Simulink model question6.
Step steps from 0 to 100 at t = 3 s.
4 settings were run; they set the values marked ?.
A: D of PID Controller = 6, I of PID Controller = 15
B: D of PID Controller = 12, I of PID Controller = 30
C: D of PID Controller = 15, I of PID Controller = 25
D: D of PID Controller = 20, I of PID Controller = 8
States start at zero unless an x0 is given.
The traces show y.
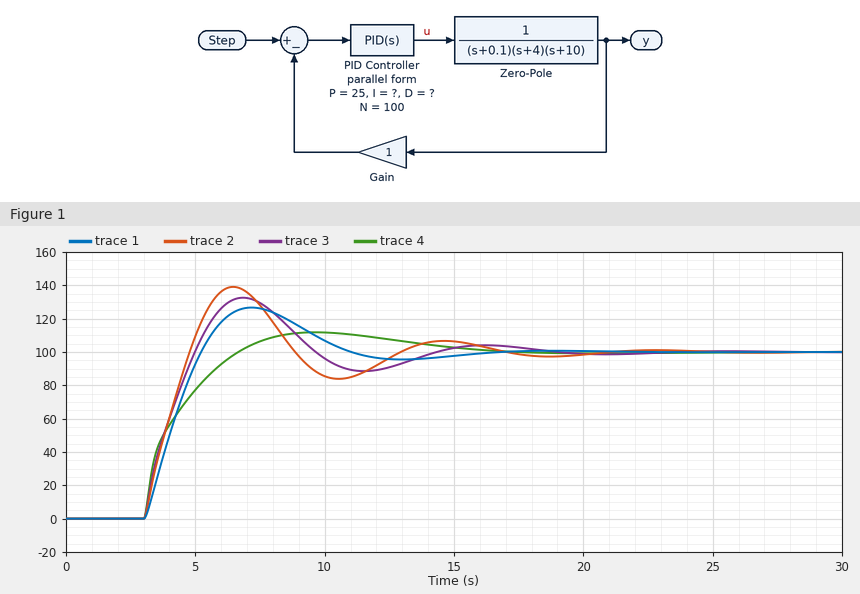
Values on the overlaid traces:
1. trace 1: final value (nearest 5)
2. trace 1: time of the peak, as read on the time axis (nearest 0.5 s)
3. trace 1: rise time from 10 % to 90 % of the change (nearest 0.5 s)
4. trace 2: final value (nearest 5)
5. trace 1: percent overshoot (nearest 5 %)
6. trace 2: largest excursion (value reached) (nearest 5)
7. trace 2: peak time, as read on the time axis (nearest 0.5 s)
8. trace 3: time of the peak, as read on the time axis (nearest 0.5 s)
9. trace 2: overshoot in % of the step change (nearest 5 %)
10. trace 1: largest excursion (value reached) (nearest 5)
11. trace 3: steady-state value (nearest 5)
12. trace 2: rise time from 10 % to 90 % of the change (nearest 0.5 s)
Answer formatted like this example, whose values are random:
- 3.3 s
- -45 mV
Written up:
- 100
- 7.0 s
- 1.5 s
- 100
- 25 %
- 140
- 6.5 s
- 7.0 s
- 40 %
- 125
- 100
- 1.5 s
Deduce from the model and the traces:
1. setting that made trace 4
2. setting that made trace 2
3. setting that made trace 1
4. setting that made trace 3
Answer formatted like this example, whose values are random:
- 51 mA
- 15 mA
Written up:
- D
- B
- A
- C
